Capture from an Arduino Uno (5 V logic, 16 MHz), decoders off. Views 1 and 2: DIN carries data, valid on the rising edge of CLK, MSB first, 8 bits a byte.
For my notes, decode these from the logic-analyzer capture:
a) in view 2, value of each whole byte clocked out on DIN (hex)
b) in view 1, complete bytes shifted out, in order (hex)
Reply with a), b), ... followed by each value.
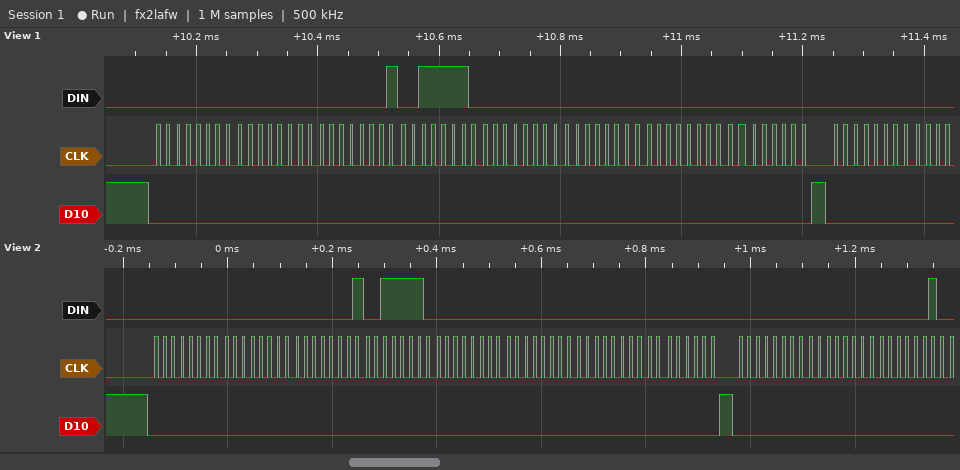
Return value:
a) 00 00 01 3E 00 00 00 00 00 00 02
b) 00 00 01 3E 00 00 00 00 00
